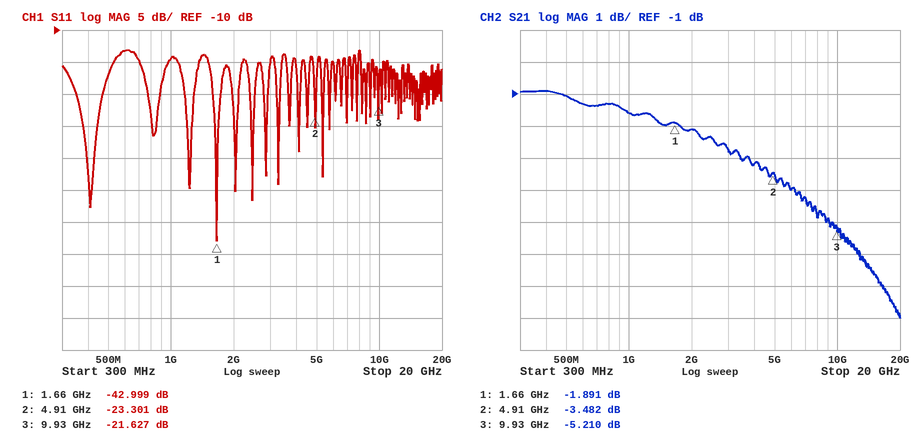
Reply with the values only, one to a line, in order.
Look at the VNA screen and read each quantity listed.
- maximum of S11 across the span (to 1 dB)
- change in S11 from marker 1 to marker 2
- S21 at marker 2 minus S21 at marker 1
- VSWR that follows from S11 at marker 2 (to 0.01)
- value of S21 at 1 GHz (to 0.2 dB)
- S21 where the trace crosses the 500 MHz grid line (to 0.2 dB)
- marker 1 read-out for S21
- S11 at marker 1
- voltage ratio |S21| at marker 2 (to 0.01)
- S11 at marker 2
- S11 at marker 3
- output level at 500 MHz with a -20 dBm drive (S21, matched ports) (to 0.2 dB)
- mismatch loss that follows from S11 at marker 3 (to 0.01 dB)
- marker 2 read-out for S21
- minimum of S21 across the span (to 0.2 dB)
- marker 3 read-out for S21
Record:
-13 dB
19.698 dB
-1.591 dB
1.15
-1.6 dB
-1.0 dB
-1.891 dB
-42.999 dB
0.67
-23.301 dB
-21.627 dB
-21.0 dBm
0.03 dB
-3.482 dB
-8.0 dB
-5.210 dB
